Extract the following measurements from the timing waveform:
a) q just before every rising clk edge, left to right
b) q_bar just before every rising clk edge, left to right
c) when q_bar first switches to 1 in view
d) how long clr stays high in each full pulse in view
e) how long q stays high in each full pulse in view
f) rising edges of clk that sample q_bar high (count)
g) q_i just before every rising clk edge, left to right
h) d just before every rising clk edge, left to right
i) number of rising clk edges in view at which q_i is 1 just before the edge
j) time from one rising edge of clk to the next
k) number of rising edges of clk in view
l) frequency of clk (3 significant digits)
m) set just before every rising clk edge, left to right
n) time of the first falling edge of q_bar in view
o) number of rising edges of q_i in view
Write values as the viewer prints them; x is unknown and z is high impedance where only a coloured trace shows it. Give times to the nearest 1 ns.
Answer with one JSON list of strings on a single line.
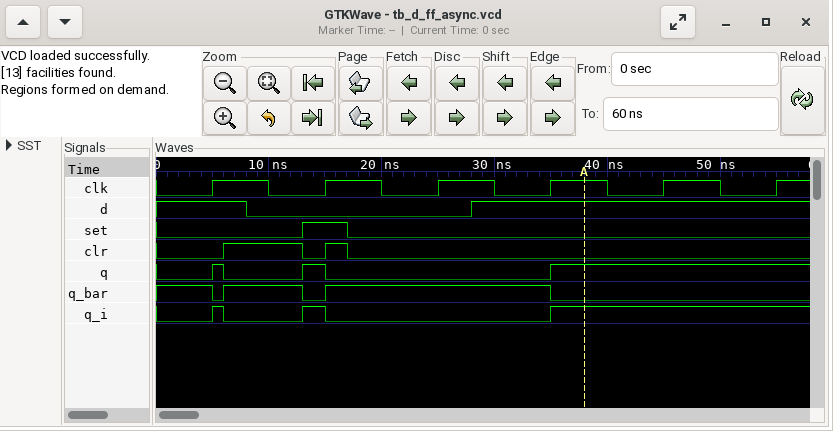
["0 1 0 0 1 1", "1 0 1 1 0 0", "6 ns", "7 ns, 2 ns", "1 ns, 2 ns", "3", "0 1 0 0 1 1", "1 0 0 1 1 1", "3", "10 ns", "6", "100 MHz", "0 1 0 0 0 0", "5 ns", "3"]
